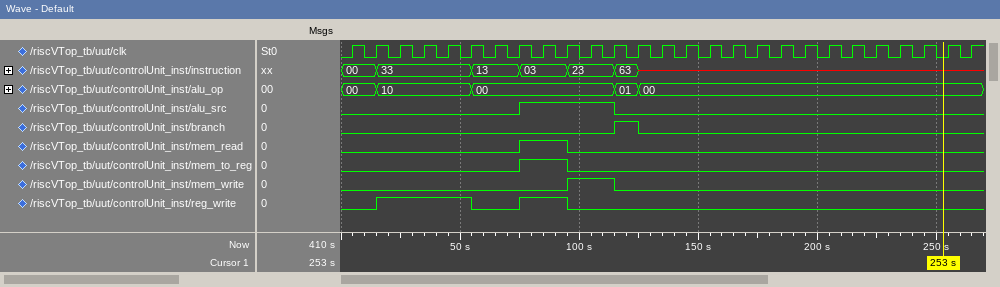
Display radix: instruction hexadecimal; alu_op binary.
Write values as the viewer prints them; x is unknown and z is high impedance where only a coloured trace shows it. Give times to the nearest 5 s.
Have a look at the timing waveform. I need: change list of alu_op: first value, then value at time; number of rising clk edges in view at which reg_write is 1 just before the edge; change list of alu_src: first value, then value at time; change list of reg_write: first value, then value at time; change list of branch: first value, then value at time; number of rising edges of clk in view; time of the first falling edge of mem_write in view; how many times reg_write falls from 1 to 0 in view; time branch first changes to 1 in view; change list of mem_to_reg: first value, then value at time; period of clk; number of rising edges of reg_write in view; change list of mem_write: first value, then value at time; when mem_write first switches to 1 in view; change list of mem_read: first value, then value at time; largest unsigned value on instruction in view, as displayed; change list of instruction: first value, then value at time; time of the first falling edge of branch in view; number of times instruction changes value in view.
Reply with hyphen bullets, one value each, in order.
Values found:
- 00, 10 at 15 s, 00 at 55 s, 01 at 115 s, 00 at 125 s
- 6
- 0, 1 at 75 s, 0 at 115 s
- 0, 1 at 15 s, 0 at 55 s, 1 at 75 s, 0 at 95 s
- 0, 1 at 115 s, 0 at 125 s
- 27
- 115 s
- 2
- 115 s
- 0, 1 at 75 s, 0 at 95 s
- 10 s
- 2
- 0, 1 at 95 s, 0 at 115 s
- 95 s
- 0, 1 at 75 s, 0 at 95 s
- 63
- 00, 33 at 15 s, 13 at 55 s, 03 at 75 s, 23 at 95 s, 63 at 115 s, x at 125 s
- 125 s
- 6
